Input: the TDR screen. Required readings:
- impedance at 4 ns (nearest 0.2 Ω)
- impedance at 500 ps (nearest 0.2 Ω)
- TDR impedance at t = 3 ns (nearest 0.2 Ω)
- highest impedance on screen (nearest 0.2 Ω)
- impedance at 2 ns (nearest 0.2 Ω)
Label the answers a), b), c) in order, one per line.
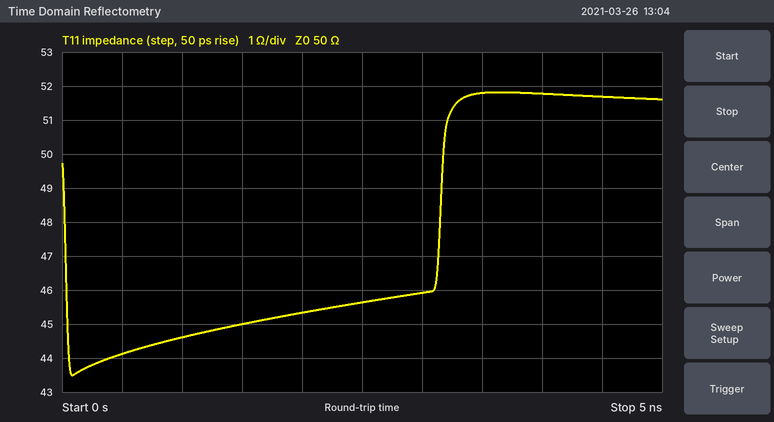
a) 51.8 Ω
b) 44.2 Ω
c) 46.0 Ω
d) 51.8 Ω
e) 45.4 Ω
